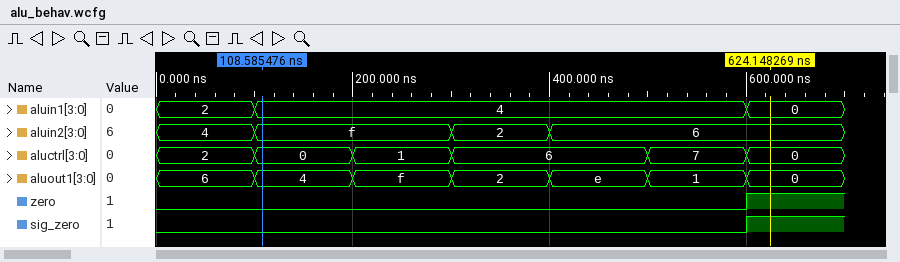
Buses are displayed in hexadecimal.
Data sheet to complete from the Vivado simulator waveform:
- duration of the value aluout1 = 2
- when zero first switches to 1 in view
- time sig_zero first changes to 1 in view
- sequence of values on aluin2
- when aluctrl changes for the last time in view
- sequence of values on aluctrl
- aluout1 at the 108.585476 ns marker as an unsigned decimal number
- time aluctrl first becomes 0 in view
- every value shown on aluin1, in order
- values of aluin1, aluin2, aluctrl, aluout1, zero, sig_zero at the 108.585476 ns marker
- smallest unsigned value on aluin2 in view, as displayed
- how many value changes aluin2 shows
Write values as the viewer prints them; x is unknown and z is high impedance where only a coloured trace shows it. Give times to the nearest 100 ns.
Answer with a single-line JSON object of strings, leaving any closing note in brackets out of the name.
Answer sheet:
{"duration of the value aluout1 = 2": "100 ns", "when zero first switches to 1 in view": "600 ns", "time sig_zero first changes to 1 in view": "600 ns", "sequence of values on aluin2": "4, f, 2, 6", "when aluctrl changes for the last time in view": "600 ns", "sequence of values on aluctrl": "2, 0, 1, 6, 7, 0", "aluout1 at the 108.585476 ns marker as an unsigned decimal number": "4", "time aluctrl first becomes 0 in view": "100 ns", "every value shown on aluin1, in order": "2, 4, 0", "values of aluin1, aluin2, aluctrl, aluout1, zero, sig_zero at the 108.585476 ns marker": "aluin1=4, aluin2=f, aluctrl=0, aluout1=4, zero=0, sig_zero=0", "smallest unsigned value on aluin2 in view, as displayed": "2", "how many value changes aluin2 shows": "3"}
